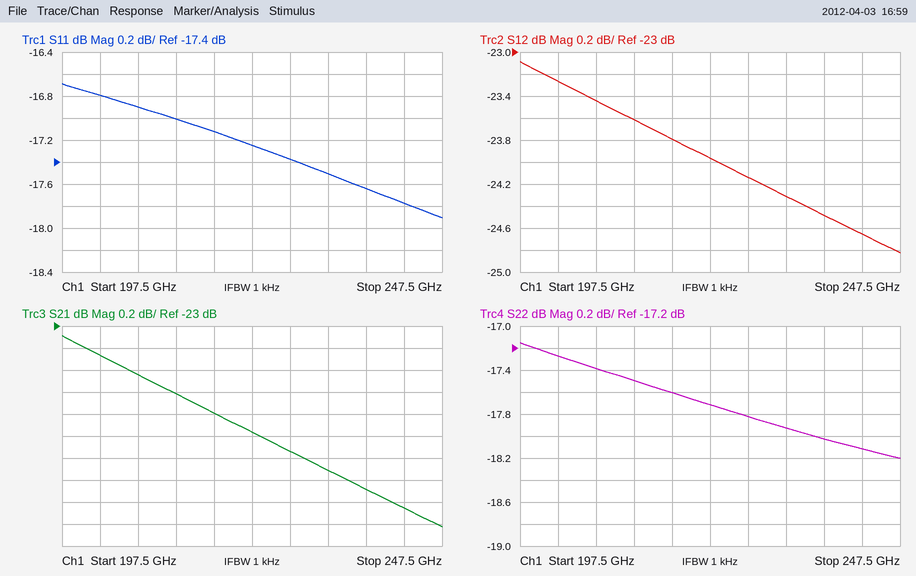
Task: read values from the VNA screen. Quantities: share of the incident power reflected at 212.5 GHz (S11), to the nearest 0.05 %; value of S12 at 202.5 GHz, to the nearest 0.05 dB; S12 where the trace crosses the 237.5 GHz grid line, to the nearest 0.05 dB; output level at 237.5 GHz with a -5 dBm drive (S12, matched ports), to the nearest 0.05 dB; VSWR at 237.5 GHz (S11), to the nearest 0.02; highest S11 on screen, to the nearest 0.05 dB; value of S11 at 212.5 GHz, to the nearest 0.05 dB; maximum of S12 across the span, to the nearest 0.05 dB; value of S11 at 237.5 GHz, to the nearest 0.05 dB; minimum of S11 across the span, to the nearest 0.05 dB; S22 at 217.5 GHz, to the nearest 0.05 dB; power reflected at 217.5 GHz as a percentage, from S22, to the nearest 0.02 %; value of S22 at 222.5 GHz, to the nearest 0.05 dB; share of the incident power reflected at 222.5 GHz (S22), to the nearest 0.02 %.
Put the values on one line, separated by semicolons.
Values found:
2.00 %; -23.25 dB; -24.50 dB; -29.50 dBm; 1.30; -16.70 dB; -17.00 dB; -23.10 dB; -17.65 dB; -17.90 dB; -17.60 dB; 1.74 %; -17.70 dB; 1.70 %
